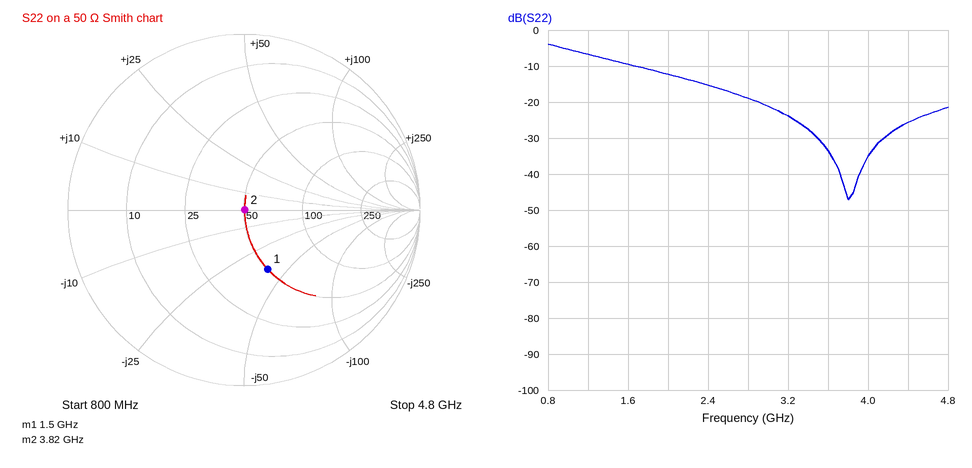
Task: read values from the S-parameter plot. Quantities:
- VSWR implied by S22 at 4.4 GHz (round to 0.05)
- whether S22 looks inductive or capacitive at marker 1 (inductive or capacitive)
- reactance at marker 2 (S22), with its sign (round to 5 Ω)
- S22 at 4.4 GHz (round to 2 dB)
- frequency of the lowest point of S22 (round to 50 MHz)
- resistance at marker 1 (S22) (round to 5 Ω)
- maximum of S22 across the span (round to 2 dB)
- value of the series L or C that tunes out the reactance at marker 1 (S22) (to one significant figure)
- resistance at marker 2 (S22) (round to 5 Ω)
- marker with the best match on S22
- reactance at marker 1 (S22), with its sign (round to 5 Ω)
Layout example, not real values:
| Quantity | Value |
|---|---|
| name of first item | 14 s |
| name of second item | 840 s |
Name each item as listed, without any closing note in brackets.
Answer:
| Quantity | Value |
|---|---|
| VSWR implied by S22 at 4.4 GHz | 1.10 |
| whether S22 looks inductive or capacitive at marker 1 | capacitive |
| reactance at marker 2 (S22), with its sign | 0 Ω |
| S22 at 4.4 GHz | -26 dB |
| frequency of the lowest point of S22 | 3.80 GHz |
| resistance at marker 1 (S22) | 50 Ω |
| maximum of S22 across the span | -4 dB |
| value of the series L or C that tunes out the reactance at marker 1 (S22) | 4 nH |
| resistance at marker 2 (S22) | 50 Ω |
| marker with the best match on S22 | marker 2 |
| reactance at marker 1 (S22), with its sign | -40 Ω |
